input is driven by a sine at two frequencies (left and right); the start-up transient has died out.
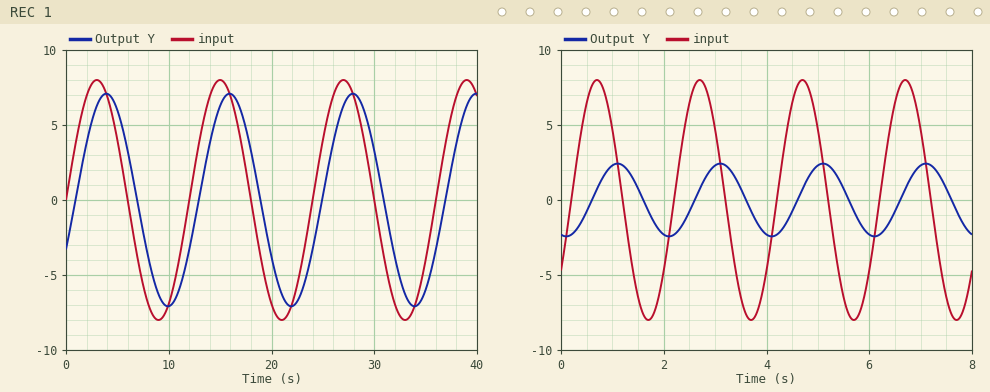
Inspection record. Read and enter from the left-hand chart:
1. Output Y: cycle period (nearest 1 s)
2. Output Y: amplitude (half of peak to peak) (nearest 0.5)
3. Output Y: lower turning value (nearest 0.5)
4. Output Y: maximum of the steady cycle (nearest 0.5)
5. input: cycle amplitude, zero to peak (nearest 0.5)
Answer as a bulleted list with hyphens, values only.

- 12 s
- 7.0
- -7.0
- 7.0
- 8.0
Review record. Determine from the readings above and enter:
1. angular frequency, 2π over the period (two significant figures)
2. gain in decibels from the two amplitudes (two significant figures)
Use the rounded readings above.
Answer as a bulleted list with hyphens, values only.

- 0.52 rad/s
- -1.2 dB
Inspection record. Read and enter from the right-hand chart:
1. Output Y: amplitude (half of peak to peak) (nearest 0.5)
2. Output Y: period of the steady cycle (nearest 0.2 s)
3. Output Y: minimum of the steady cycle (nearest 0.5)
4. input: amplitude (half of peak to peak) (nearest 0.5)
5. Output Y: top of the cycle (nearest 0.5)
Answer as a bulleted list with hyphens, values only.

- 2.5
- 2.0 s
- -2.5
- 8.0
- 2.5
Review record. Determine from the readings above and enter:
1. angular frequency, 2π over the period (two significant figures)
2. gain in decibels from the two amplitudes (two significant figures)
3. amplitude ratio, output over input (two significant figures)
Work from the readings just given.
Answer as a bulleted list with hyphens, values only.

- 3.1 rad/s
- -10 dB
- 0.31
